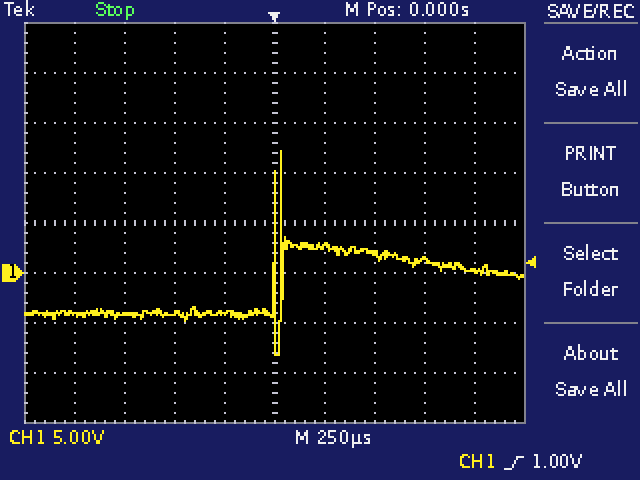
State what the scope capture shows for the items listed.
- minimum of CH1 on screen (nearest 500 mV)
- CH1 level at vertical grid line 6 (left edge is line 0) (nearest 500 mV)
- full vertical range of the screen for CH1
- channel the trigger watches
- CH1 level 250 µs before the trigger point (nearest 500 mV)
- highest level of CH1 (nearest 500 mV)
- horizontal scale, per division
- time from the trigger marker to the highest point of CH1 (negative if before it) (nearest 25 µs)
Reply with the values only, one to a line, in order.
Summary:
-8.0 V
2.5 V
40 V
CH1
-4.0 V
12.0 V
250 µs
+25 µs
